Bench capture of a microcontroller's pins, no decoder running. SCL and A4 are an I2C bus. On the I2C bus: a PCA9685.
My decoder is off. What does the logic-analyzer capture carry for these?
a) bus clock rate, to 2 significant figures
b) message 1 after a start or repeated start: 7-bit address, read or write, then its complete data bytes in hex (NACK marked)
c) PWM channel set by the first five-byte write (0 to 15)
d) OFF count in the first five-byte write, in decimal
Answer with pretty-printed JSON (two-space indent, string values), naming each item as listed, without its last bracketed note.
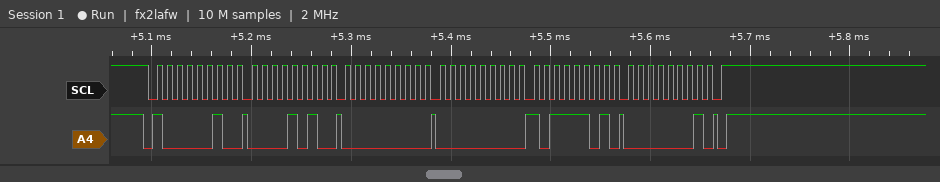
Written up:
{
  "bus clock rate, to 2 significant figures": "100 kHz",
  "message 1 after a start or repeated start: 7-bit address, read or write, then its complete data bytes in hex": "0x41 write: 0A 00 00 BD 01",
  "PWM channel set by the first five-byte write": "1",
  "OFF count in the first five-byte write, in decimal": "445"
}
